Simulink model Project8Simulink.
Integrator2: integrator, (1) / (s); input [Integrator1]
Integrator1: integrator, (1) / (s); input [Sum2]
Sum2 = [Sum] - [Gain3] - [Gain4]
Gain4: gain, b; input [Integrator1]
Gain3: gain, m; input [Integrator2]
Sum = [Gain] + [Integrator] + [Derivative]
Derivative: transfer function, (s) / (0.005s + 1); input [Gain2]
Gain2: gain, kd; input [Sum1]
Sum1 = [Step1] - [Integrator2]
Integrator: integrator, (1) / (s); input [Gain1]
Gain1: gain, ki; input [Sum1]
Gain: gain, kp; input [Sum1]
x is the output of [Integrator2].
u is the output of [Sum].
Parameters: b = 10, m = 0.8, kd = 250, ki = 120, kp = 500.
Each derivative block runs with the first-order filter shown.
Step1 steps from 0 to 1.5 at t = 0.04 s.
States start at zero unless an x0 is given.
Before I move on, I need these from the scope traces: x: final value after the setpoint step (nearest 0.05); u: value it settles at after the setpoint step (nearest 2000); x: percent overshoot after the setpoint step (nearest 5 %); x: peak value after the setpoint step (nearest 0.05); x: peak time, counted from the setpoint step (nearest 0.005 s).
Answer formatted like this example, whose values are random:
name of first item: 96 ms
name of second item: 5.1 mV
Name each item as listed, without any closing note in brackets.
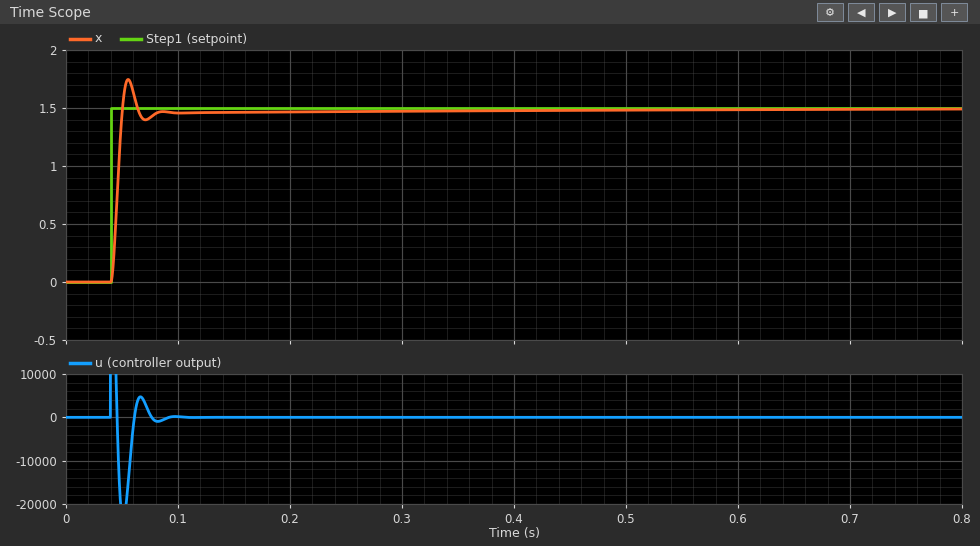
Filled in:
x: final value after the setpoint step: 1.50
u: value it settles at after the setpoint step: 0
x: percent overshoot after the setpoint step: 15 %
x: peak value after the setpoint step: 1.75
x: peak time, counted from the setpoint step: 0.015 s
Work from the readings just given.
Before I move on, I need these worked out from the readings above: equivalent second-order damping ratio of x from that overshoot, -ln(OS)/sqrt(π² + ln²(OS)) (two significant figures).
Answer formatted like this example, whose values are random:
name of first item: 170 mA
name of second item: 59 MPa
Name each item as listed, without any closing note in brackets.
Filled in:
equivalent second-order damping ratio of x from that overshoot, -ln(OS)/sqrt(π² + ln²(OS)): 0.52
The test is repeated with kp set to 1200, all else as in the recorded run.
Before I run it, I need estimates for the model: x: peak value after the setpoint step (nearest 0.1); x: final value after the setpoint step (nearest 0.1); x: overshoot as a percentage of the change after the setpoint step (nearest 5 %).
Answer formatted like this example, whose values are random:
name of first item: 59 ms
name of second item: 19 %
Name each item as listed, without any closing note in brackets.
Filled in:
x: peak value after the setpoint step: 1.8
x: final value after the setpoint step: 1.5
x: overshoot as a percentage of the change after the setpoint step: 20 %
